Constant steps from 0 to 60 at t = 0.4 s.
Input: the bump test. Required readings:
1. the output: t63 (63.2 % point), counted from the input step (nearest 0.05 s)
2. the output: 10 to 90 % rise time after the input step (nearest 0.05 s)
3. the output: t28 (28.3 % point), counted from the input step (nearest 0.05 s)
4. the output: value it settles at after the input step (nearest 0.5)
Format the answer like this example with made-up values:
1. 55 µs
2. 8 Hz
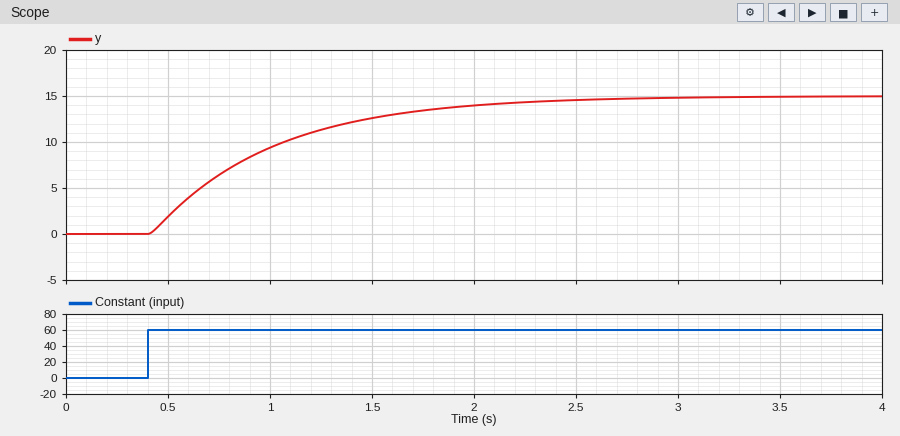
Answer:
1. 0.60 s
2. 1.30 s
3. 0.20 s
4. 15.0
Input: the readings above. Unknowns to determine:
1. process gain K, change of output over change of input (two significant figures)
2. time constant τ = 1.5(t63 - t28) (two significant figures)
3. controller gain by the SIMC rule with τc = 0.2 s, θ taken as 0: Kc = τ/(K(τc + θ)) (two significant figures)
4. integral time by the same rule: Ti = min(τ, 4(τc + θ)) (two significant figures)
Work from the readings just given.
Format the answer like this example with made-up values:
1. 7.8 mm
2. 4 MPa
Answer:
1. 0.25
2. 0.60 s
3. 12
4. 0.60 s
